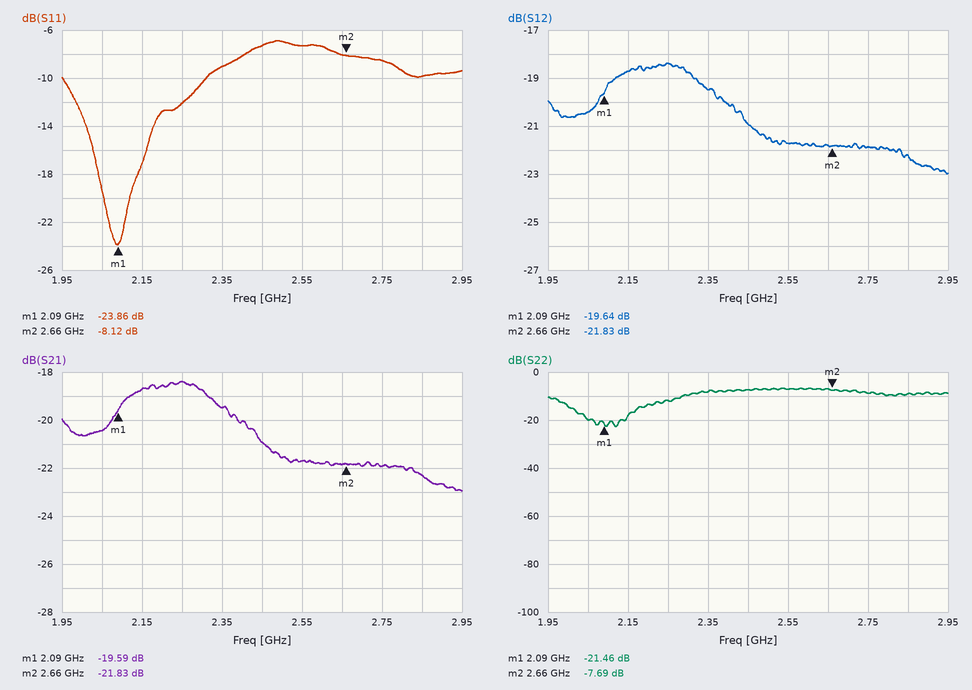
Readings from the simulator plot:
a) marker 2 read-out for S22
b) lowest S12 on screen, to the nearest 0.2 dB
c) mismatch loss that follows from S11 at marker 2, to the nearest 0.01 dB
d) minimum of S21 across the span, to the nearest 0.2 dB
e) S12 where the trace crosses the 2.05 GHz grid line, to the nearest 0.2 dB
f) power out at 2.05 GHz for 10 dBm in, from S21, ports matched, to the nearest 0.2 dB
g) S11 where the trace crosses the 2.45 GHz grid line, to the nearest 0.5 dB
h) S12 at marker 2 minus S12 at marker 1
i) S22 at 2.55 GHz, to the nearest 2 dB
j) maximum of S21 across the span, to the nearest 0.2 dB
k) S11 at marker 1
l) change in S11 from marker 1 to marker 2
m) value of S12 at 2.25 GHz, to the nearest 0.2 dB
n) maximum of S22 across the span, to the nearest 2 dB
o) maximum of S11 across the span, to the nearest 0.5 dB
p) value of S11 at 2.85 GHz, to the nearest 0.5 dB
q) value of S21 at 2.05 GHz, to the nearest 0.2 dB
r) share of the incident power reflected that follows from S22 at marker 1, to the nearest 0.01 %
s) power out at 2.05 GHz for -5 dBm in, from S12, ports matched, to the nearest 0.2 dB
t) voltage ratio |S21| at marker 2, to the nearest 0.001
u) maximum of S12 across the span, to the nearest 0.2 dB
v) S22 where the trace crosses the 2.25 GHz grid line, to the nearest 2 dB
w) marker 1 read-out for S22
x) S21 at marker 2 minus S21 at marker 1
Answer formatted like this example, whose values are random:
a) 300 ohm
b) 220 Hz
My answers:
a) -7.69 dB
b) -23.0 dB
c) 0.73 dB
d) -23.0 dB
e) -20.4 dB
f) -10.4 dBm
g) -7.5 dB
h) -2.19 dB
i) -8 dB
j) -18.4 dB
k) -23.86 dB
l) 15.74 dB
m) -18.4 dB
n) -6 dB
o) -7.0 dB
p) -10.0 dB
q) -20.4 dB
r) 0.71 %
s) -25.4 dBm
t) 0.081
u) -18.4 dB
v) -12 dB
w) -21.46 dB
x) -2.24 dB
